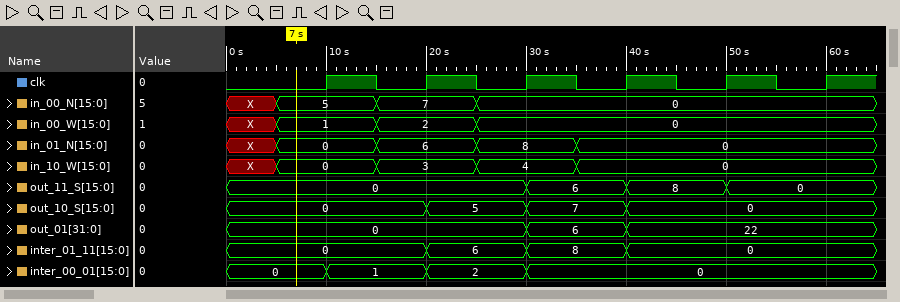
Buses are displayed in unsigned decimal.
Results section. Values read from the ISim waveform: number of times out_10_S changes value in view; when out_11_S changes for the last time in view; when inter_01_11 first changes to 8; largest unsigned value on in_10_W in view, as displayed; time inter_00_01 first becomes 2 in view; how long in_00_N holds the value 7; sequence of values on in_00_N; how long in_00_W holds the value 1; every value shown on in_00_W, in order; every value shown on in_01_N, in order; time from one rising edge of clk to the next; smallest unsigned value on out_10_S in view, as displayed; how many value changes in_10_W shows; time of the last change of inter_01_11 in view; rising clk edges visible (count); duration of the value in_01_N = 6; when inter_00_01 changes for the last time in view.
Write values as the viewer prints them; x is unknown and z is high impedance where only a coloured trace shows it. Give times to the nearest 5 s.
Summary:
3
50 s
30 s
4
20 s
10 s
X, 5, 7, 0
10 s
X, 1, 2, 0
X, 0, 6, 8, 0
10 s
0
4
40 s
6
10 s
30 s
